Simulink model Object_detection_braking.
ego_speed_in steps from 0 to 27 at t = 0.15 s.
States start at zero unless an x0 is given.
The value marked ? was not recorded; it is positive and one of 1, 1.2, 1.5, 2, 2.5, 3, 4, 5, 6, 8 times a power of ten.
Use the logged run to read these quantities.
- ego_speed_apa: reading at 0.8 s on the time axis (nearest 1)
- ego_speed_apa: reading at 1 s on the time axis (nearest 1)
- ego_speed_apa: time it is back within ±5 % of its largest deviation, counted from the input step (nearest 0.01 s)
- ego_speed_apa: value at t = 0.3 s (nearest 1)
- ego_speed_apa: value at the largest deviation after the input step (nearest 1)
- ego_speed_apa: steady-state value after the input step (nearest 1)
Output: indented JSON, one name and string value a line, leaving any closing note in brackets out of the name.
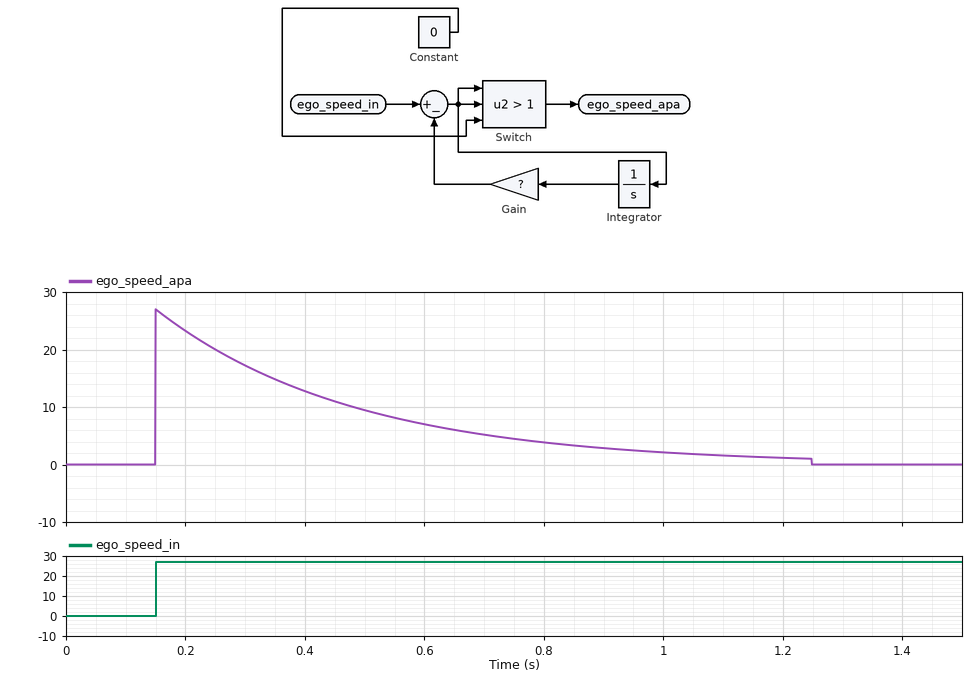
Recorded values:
{
  "ego_speed_apa: reading at 0.8 s on the time axis": "4",
  "ego_speed_apa: reading at 1 s on the time axis": "2",
  "ego_speed_apa: time it is back within ±5 % of its largest deviation, counted from the input step": "1.00 s",
  "ego_speed_apa: value at t = 0.3 s": "17",
  "ego_speed_apa: value at the largest deviation after the input step": "27",
  "ego_speed_apa: steady-state value after the input step": "0"
}
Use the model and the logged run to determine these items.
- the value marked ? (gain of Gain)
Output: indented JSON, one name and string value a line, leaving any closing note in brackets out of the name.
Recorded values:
{
  "the value marked ?": "3"
}
